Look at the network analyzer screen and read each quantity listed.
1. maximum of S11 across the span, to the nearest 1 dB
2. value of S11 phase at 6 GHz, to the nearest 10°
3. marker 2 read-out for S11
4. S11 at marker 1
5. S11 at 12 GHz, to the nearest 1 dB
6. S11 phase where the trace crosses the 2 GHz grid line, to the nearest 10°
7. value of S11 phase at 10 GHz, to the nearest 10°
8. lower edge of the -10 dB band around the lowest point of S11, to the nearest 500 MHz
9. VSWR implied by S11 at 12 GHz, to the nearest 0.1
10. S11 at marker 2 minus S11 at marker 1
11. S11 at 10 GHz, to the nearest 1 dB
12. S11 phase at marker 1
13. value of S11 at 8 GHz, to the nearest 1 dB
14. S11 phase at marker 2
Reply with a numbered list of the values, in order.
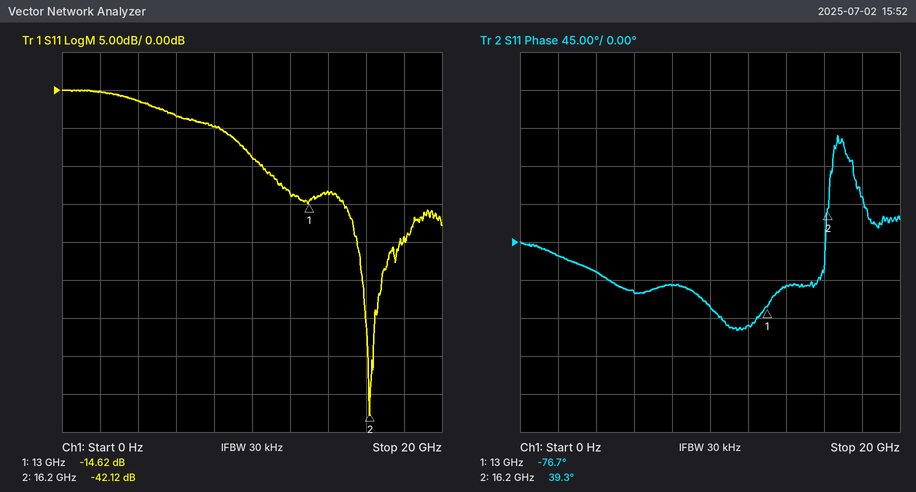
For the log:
1. 0 dB
2. -60°
3. -42.12 dB
4. -14.62 dB
5. -14 dB
6. -20°
7. -80°
8. 10.5 GHz
9. 1.5
10. -27.50 dB
11. -9 dB
12. -76.7°
13. -5 dB
14. 39.3°
